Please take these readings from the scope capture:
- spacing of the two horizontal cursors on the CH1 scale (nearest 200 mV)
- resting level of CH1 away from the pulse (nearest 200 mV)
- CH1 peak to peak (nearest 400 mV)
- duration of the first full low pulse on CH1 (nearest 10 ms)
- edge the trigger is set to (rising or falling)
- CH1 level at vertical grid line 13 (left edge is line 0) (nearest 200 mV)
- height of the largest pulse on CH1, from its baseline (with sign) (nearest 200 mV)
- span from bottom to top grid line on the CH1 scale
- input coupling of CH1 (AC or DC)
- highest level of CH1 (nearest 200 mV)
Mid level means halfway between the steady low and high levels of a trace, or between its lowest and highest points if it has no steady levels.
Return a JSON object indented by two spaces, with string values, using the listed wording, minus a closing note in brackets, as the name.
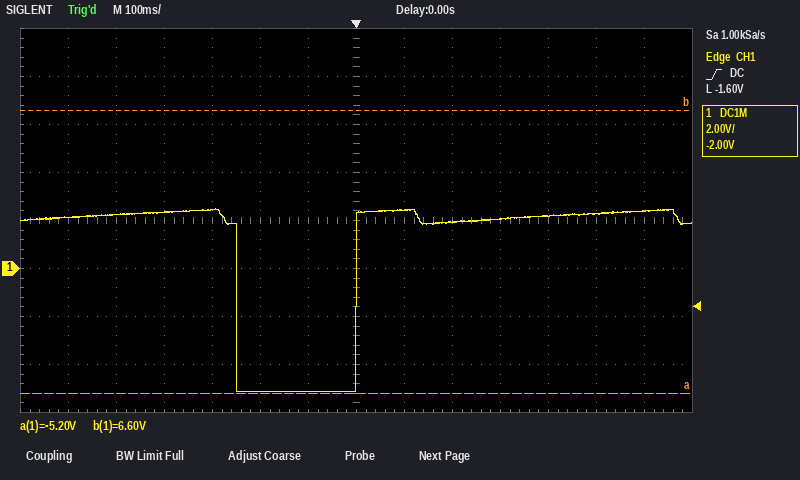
{
  "spacing of the two horizontal cursors on the CH1 scale": "11.8 V",
  "resting level of CH1 away from the pulse": "2.2 V",
  "CH1 peak to peak": "7.6 V",
  "duration of the first full low pulse on CH1": "250 ms",
  "edge the trigger is set to": "rising",
  "CH1 level at vertical grid line 13 (left edge is line 0)": "2.4 V",
  "height of the largest pulse on CH1, from its baseline (with sign)": "-7.4 V",
  "span from bottom to top grid line on the CH1 scale": "16 V",
  "input coupling of CH1": "DC",
  "highest level of CH1": "2.4 V"
}
